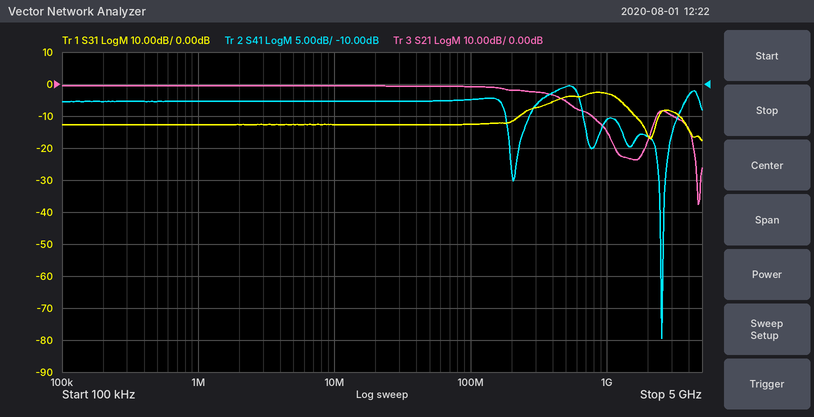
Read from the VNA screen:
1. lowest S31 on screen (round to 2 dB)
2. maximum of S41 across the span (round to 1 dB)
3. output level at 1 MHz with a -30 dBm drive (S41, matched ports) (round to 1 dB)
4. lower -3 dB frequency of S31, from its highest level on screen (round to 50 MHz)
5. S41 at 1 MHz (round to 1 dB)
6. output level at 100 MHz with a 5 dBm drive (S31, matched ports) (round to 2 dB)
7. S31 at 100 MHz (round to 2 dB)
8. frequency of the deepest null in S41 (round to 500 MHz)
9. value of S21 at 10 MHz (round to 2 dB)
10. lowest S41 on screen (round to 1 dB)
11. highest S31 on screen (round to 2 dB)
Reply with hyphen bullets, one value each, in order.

- -18 dB
- -10 dB
- -43 dBm
- 400 MHz
- -13 dB
- -8 dBm
- -12 dB
- 2.5 GHz
- 0 dB
- -50 dB
- -2 dB
